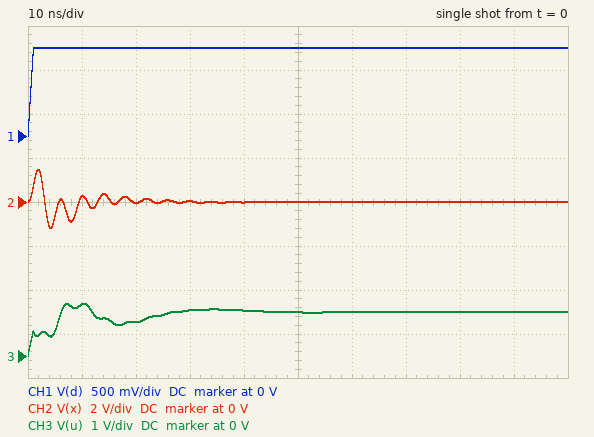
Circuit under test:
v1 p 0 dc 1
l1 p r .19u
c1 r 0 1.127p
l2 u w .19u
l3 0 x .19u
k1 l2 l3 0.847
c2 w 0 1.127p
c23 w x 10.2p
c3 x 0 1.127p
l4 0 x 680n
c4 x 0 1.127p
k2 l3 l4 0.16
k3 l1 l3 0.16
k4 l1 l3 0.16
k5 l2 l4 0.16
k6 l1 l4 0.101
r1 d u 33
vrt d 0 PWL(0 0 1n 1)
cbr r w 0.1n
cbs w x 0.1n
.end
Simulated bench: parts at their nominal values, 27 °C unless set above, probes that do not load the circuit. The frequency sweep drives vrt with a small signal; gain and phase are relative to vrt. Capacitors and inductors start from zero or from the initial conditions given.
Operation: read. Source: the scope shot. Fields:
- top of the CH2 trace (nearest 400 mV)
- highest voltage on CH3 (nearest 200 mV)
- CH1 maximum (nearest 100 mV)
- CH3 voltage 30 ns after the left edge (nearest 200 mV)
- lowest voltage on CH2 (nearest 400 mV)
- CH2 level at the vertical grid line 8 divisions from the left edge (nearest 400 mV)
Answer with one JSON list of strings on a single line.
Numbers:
["1.6 V", "1.2 V", "1.0 V", "1.0 V", "-1.2 V", "0 V"]
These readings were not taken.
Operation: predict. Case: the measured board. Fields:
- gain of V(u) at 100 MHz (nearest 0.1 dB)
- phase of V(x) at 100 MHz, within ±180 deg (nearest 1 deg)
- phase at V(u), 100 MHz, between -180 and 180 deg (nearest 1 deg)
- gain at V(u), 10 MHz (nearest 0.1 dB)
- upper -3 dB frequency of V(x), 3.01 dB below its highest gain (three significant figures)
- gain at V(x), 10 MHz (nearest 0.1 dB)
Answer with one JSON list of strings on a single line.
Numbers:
["-8.8 dB", "69 deg", "69 deg", "-1.0 dB", "270 MHz", "-31.1 dB"]
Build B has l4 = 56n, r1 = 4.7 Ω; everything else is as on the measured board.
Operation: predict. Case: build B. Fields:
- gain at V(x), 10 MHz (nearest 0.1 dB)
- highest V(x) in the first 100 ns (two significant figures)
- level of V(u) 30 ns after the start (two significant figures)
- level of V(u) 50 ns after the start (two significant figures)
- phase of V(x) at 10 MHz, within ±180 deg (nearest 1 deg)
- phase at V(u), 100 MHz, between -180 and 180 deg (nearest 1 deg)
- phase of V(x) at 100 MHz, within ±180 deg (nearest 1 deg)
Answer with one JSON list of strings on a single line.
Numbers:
["-41.0 dB", "740 mV", "990 mV", "960 mV", "-4 deg", "-57 deg", "123 deg"]
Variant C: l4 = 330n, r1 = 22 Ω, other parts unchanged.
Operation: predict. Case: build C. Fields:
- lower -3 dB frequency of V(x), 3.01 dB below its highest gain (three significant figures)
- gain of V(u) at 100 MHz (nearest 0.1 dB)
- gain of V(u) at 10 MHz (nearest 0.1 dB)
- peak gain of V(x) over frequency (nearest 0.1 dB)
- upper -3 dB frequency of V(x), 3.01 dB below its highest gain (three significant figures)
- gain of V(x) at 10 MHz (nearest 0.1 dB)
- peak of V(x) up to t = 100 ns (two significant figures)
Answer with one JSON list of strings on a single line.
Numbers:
["254 MHz", "-8.3 dB", "-0.5 dB", "18.1 dB", "278 MHz", "-32.2 dB", "1.4 V"]
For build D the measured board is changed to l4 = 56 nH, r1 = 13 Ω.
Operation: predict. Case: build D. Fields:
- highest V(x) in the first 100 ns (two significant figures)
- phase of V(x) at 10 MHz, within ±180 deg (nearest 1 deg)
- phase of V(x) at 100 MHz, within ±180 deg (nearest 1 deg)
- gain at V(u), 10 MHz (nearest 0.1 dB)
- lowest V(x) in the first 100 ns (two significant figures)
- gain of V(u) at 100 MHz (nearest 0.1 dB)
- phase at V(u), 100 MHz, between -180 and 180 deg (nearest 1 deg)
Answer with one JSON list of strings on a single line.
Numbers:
["690 mV", "-11 deg", "103 deg", "-0.2 dB", "-680 mV", "-12.8 dB", "-77 deg"]
